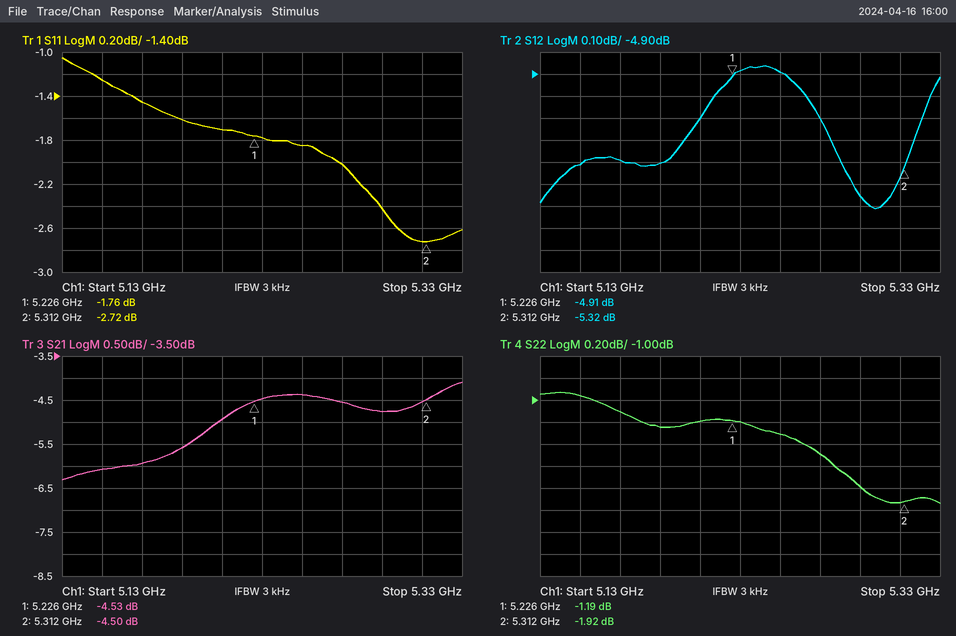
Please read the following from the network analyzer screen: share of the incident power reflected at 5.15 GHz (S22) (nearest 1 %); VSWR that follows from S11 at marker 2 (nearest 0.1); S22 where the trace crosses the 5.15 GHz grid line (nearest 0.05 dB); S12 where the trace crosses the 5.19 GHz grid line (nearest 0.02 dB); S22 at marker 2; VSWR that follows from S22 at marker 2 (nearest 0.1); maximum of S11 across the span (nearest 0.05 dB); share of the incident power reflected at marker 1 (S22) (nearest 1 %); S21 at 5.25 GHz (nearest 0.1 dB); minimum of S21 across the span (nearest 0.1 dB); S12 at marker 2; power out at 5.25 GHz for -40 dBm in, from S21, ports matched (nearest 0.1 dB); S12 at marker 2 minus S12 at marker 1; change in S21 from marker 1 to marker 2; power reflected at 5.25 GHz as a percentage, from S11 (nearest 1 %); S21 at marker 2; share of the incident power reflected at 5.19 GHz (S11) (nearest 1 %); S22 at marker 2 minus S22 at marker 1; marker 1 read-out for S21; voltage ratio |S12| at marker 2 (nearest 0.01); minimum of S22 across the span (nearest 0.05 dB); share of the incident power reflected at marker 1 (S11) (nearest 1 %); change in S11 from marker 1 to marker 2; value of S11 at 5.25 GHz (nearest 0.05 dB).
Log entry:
80 %
6.4
-0.95 dB
-5.30 dB
-1.92 dB
9.1
-1.05 dB
76 %
-4.4 dB
-6.3 dB
-5.32 dB
-44.4 dBm
-0.41 dB
0.03 dB
65 %
-4.50 dB
69 %
-0.73 dB
-4.53 dB
0.54
-1.95 dB
67 %
-0.96 dB
-1.85 dB
